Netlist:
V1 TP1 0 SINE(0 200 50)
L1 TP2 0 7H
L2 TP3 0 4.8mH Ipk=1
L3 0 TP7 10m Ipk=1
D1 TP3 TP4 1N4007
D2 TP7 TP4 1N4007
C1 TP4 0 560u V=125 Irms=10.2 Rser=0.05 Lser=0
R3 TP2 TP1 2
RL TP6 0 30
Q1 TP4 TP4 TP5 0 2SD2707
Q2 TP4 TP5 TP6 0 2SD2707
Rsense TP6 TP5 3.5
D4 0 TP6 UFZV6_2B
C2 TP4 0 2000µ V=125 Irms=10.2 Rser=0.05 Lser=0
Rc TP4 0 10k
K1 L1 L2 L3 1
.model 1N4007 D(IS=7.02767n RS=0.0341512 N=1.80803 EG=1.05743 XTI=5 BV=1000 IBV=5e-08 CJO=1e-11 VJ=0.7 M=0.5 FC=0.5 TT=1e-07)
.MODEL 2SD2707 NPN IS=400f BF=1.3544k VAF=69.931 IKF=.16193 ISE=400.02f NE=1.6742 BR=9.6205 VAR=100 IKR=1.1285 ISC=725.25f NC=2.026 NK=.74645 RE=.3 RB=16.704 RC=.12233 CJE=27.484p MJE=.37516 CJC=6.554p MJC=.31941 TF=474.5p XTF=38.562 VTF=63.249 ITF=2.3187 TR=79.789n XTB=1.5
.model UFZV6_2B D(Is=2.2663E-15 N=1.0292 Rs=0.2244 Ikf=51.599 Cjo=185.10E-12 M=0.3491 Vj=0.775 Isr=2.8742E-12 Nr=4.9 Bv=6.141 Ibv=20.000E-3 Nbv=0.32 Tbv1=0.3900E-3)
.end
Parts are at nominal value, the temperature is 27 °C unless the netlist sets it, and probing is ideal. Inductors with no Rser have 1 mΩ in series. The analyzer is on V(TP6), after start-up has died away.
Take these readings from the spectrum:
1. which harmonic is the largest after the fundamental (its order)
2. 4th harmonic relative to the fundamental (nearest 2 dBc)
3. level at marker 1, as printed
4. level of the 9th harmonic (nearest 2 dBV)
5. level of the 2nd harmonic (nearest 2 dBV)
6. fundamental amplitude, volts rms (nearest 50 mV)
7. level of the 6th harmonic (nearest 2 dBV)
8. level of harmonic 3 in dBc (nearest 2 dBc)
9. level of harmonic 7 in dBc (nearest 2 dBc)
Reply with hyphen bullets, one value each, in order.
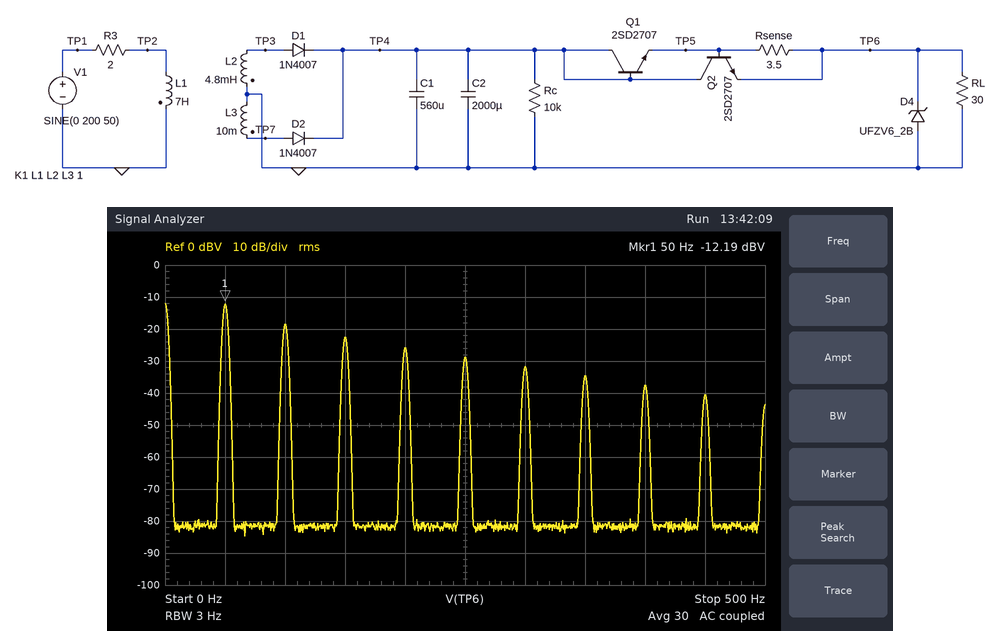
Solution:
- 2
- -14 dBc
- -12.19 dBV
- -40 dBV
- -18 dBV
- 250 mV
- -32 dBV
- -10 dBc
- -22 dBc
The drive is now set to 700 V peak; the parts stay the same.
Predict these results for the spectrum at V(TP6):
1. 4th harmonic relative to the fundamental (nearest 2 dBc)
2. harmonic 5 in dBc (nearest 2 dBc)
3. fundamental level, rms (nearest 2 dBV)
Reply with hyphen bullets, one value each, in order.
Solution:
- -18 dBc
- -20 dBc
- -22 dBV
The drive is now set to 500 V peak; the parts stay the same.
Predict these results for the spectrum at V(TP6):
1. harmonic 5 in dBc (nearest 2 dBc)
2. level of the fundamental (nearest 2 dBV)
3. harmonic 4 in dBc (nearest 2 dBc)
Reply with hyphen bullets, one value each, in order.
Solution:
- -20 dBc
- -24 dBV
- -18 dBc
